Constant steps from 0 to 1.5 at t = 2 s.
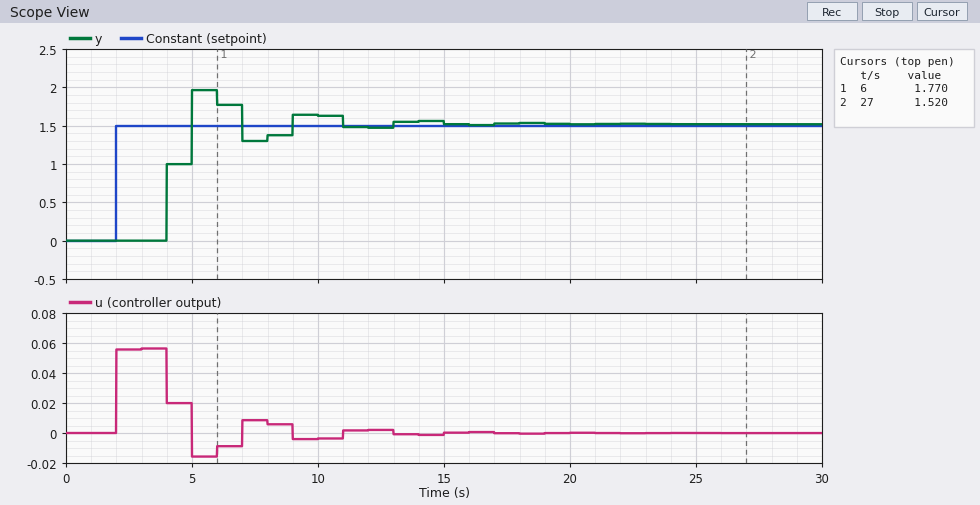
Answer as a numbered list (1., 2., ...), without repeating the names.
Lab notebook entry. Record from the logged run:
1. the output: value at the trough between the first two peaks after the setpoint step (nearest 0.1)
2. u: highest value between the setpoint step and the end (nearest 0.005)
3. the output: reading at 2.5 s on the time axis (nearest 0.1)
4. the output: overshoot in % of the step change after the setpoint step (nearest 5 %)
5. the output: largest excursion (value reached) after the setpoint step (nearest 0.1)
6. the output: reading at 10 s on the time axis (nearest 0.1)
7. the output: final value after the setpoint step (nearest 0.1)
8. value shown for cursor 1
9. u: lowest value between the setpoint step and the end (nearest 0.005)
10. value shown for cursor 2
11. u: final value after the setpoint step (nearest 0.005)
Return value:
1. 1.3
2. 0.055
3. 0.0
4. 30 %
5. 2.0
6. 1.6
7. 1.5
8. 1.770
9. -0.015
10. 1.520
11. 0.000
